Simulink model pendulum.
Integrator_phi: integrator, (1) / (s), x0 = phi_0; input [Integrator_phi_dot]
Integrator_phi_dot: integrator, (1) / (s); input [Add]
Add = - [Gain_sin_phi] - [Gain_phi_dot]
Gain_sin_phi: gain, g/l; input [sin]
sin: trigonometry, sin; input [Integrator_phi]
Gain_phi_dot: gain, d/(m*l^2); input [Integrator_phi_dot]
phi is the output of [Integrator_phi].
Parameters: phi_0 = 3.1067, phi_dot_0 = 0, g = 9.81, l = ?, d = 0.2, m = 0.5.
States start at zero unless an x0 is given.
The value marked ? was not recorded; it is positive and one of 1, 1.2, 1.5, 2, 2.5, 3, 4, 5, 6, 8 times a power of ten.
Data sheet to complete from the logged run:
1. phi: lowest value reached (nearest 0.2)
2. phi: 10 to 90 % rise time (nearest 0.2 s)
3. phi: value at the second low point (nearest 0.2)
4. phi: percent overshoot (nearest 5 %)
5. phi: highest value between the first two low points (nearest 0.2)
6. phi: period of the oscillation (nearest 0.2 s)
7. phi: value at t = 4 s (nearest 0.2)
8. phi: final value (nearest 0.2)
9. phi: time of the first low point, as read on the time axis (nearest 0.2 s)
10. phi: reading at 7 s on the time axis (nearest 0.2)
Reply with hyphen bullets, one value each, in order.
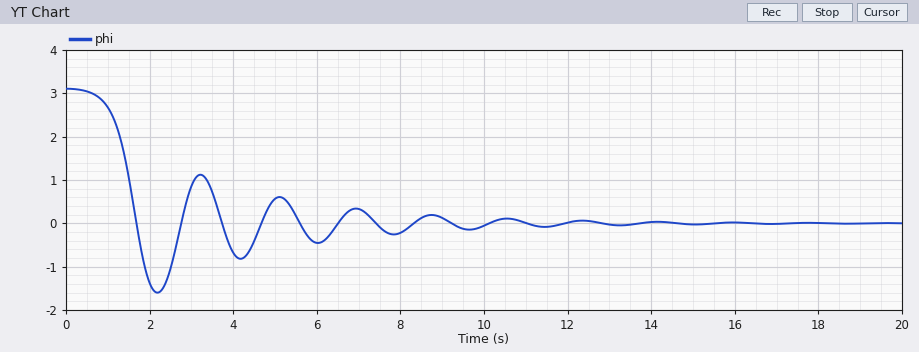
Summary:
- -1.6
- 0.8 s
- -0.8
- 50 %
- 1.2
- 2.0 s
- -0.6
- 0.0
- 2.2 s
- 0.4
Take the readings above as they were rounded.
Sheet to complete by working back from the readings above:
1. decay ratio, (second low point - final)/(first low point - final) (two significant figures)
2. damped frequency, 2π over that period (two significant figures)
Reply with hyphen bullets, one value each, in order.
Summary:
- 0.50
- 3.1 rad/s
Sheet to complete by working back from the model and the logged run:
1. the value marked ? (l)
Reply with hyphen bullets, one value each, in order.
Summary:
- 0.8
